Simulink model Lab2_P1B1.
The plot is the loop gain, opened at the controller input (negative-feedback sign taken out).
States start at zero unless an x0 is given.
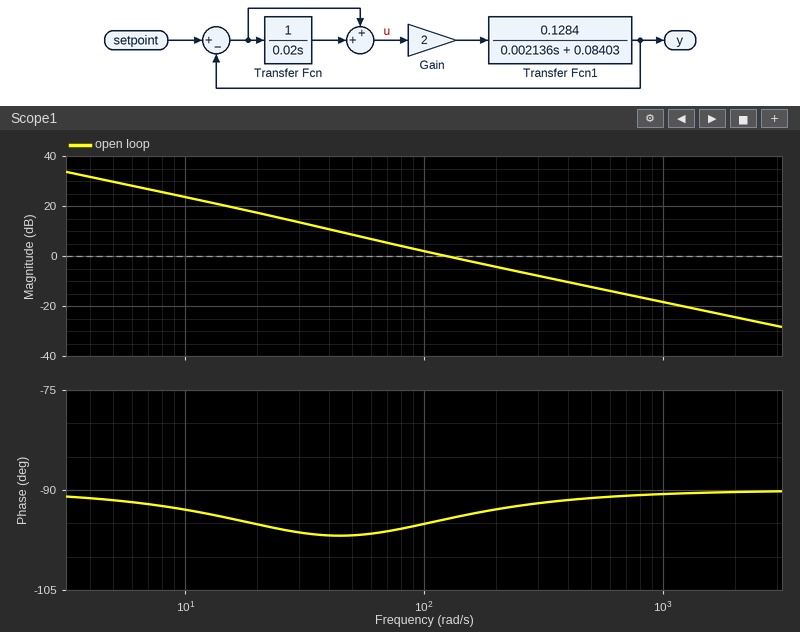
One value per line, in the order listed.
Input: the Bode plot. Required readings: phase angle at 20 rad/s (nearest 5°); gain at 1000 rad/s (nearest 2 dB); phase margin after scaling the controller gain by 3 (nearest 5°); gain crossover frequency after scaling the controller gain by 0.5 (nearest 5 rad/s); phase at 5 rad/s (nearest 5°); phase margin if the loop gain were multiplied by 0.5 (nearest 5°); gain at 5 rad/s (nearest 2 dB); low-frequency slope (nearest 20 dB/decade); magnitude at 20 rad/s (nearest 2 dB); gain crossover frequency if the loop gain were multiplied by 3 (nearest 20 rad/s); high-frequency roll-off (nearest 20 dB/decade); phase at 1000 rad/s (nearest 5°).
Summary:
-95°
-18 dB
90°
65 rad/s
-90°
85°
30 dB
-20 dB/decade
18 dB
360 rad/s
-20 dB/decade
-90°
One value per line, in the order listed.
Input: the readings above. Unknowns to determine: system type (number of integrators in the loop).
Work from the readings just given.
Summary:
1
